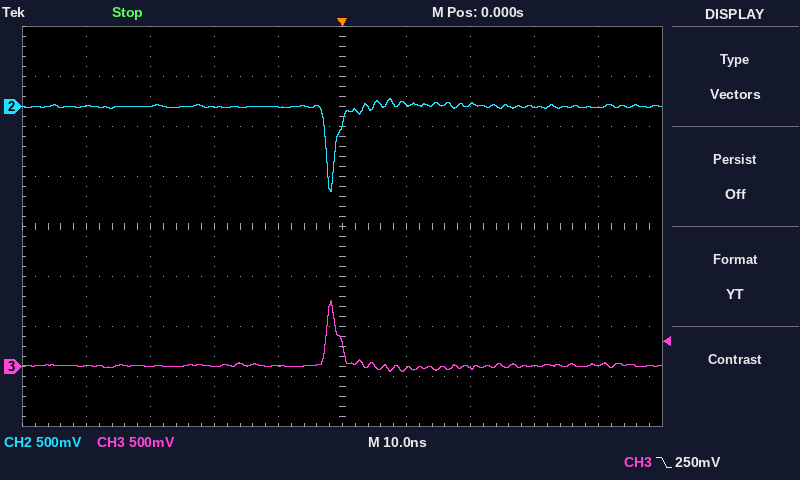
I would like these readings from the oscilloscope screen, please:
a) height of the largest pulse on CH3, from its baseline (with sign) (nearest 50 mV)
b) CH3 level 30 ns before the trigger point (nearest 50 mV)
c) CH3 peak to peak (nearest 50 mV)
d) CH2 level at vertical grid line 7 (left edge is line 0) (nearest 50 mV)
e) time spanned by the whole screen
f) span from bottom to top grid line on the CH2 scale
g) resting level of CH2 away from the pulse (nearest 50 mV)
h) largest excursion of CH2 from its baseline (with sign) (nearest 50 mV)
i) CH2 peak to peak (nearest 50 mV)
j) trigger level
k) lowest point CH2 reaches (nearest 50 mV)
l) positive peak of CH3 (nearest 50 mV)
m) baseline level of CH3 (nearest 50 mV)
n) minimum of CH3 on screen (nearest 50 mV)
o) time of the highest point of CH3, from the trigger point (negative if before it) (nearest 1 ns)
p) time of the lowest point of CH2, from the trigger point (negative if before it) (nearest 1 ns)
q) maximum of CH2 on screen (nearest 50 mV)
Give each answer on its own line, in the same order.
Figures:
+650 mV
0 mV
700 mV
0 mV
100 ns
4 V
0 mV
-850 mV
950 mV
250 mV
-850 mV
650 mV
0 mV
-50 mV
-2 ns
-2 ns
100 mV
